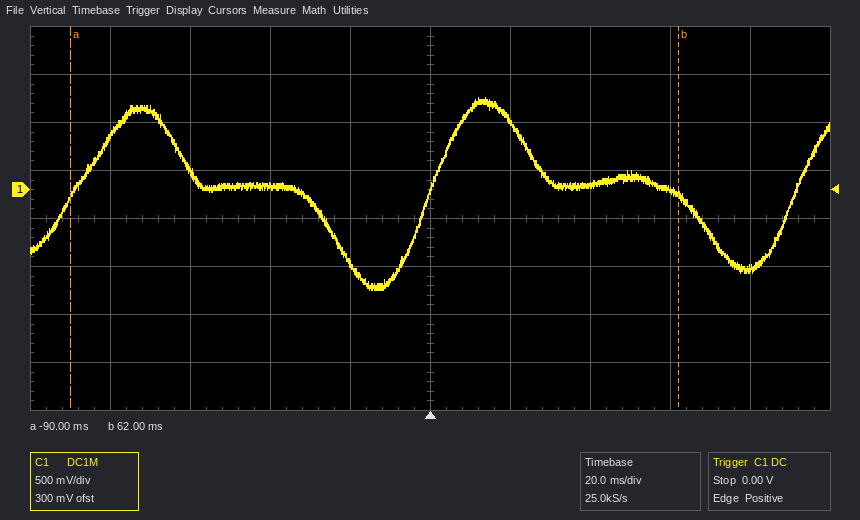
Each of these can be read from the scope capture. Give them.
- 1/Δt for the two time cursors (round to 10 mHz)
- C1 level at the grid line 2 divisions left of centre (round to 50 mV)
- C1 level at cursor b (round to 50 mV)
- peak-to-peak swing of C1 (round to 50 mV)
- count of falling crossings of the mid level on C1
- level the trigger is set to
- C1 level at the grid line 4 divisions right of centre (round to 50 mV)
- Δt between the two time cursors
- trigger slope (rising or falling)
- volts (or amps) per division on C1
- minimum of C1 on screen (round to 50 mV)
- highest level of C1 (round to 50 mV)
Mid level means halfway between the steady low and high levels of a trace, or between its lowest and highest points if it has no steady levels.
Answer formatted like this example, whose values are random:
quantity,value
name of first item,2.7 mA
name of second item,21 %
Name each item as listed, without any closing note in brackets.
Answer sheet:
quantity,value
1/Δt for the two time cursors,6.58 Hz
C1 level at the grid line 2 divisions left of centre,50 mV
C1 level at cursor b,-50 mV
peak-to-peak swing of C1,2.00 V
count of falling crossings of the mid level on C1,2
level the trigger is set to,0.00 V
C1 level at the grid line 4 divisions right of centre,-800 mV
Δt between the two time cursors,152 ms
trigger slope,rising
volts (or amps) per division on C1,500 mV
minimum of C1 on screen,-1.05 V
highest level of C1,950 mV
